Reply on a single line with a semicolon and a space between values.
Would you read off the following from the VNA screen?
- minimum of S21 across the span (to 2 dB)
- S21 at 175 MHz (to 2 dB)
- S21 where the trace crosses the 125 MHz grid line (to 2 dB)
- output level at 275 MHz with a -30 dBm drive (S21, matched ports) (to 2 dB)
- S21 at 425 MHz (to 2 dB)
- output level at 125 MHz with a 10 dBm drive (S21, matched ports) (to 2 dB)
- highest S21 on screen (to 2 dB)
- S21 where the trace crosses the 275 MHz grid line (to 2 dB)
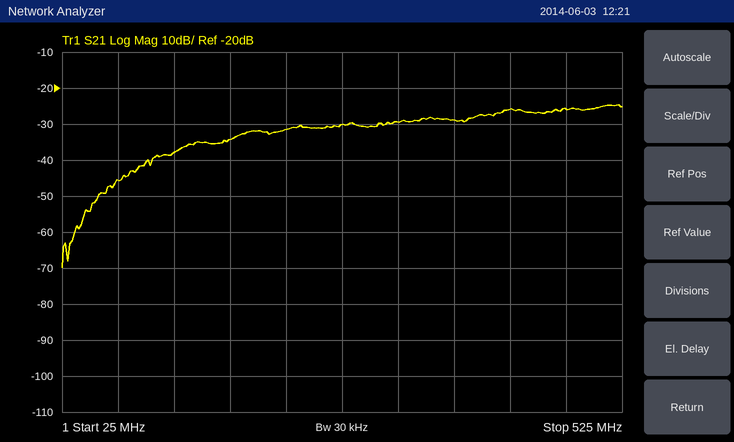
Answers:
-70 dB; -34 dB; -38 dB; -60 dBm; -26 dB; -28 dBm; -24 dB; -30 dB
